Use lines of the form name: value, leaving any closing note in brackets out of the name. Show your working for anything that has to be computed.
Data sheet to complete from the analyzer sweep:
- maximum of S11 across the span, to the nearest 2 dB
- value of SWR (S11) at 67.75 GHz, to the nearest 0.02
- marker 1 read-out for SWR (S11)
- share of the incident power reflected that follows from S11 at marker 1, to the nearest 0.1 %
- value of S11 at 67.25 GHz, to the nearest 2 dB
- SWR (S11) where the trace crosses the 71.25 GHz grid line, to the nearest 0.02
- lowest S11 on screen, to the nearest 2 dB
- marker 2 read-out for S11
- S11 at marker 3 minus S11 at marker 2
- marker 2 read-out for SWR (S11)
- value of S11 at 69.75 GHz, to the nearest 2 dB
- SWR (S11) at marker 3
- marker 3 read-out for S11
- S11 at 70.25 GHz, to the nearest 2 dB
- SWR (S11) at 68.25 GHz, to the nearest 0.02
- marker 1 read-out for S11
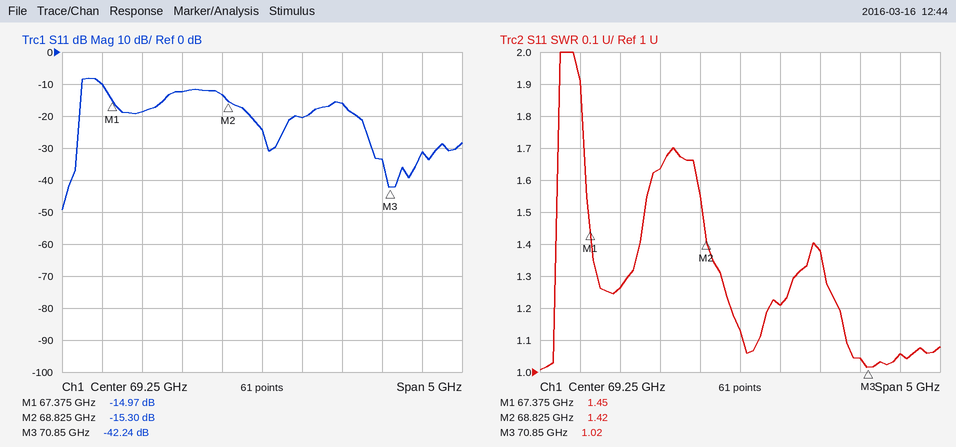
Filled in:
maximum of S11 across the span, to the nearest 2 dB: -8 dB
value of SWR (S11) at 67.75 GHz, to the nearest 0.02: 1.26
marker 1 read-out for SWR: 1.45
share of the incident power reflected that follows from S11 at marker 1, to the nearest 0.1 %: 10^(-14.97/10) ≈ 3.2 %
value of S11 at 67.25 GHz, to the nearest 2 dB: -10 dB
SWR (S11) where the trace crosses the 71.25 GHz grid line, to the nearest 0.02: 1.06
lowest S11 on screen, to the nearest 2 dB: -50 dB
marker 2 read-out for S11: -15.30 dB
S11 at marker 3 minus S11 at marker 2: -42.24 − (-15.3) = -26.94 dB
marker 2 read-out for SWR: 1.42
value of S11 at 69.75 GHz, to the nearest 2 dB: -20 dB
SWR (S11) at marker 3: 1.02
marker 3 read-out for S11: -42.24 dB
S11 at 70.25 GHz, to the nearest 2 dB: -16 dB
SWR (S11) at 68.25 GHz, to the nearest 0.02: 1.64
marker 1 read-out for S11: -14.97 dB
